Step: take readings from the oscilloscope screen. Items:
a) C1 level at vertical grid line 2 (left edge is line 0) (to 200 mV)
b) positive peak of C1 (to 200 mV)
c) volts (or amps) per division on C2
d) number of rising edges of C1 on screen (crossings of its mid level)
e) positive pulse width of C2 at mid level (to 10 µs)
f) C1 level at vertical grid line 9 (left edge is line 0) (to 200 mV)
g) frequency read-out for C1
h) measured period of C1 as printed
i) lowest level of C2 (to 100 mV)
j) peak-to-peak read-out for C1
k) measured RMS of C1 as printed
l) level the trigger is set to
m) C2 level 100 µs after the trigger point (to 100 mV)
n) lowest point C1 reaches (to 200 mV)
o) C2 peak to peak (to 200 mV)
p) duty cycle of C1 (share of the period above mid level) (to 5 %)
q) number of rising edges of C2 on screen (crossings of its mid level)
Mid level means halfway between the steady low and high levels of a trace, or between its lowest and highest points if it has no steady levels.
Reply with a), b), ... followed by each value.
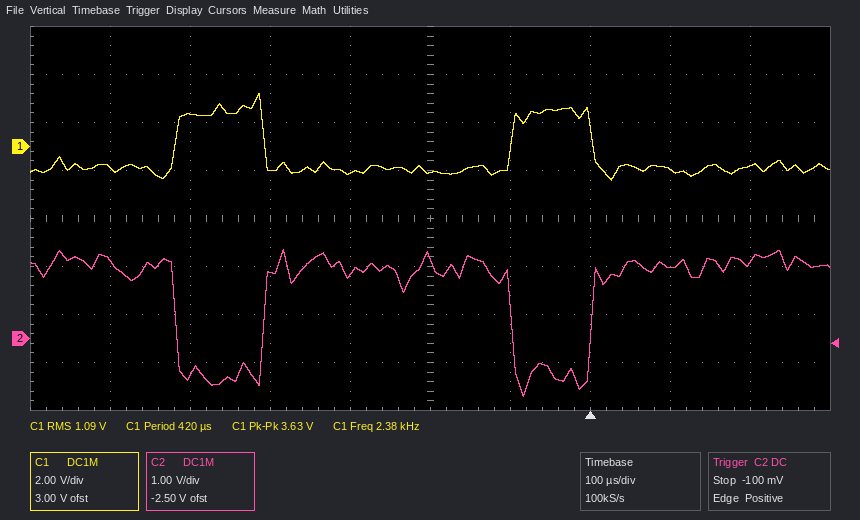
a) 1.4 V
b) 2.2 V
c) 1 V
d) 2
e) 310 µs
f) -800 mV
g) 2.38 kHz
h) 420 µs
i) -1.2 V
j) 3.63 V
k) 1.09 V
l) -100 mV
m) 1.5 V
n) -1.4 V
o) 3.0 V
p) 25 %
q) 2
